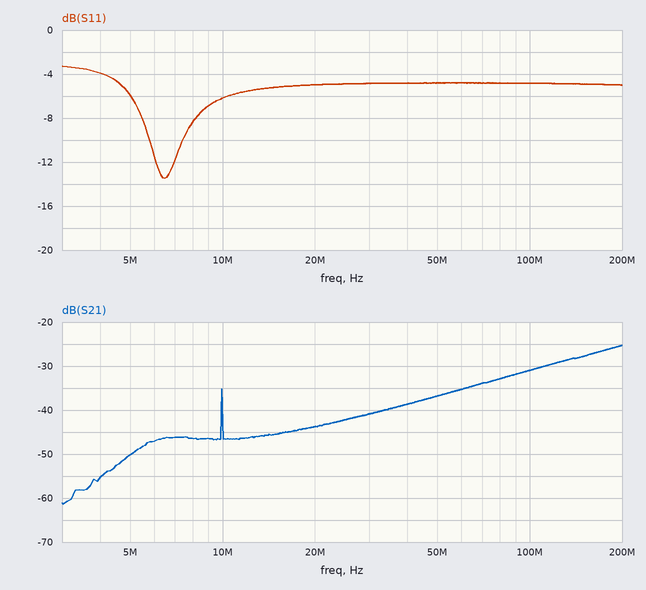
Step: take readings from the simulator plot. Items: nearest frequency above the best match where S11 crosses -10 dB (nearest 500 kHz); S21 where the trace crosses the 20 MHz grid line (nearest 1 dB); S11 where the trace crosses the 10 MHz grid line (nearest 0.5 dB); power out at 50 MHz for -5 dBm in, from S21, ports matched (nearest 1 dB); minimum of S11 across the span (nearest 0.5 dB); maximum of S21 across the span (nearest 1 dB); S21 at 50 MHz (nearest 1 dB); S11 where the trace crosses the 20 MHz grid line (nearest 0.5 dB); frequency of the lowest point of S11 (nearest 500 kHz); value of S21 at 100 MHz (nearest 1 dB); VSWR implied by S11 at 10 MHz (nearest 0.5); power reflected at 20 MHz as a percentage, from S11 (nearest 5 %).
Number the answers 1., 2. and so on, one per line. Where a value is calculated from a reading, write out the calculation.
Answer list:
1. 7.5 MHz
2. -44 dB
3. -6.0 dB
4. -5 dBm + (-37 dB) = -42 dBm
5. -13.5 dB
6. -25 dB
7. -37 dB
8. -5.0 dB
9. 6.5 MHz
10. -31 dB
11. |Γ| = 10^(-6/20) = 0.5012; VSWR = (1 + 0.5012)/(1 − 0.5012) ≈ 3.0
12. 10^(-5/10) ≈ 31.6 %, so 30 % to the nearest 5 %
